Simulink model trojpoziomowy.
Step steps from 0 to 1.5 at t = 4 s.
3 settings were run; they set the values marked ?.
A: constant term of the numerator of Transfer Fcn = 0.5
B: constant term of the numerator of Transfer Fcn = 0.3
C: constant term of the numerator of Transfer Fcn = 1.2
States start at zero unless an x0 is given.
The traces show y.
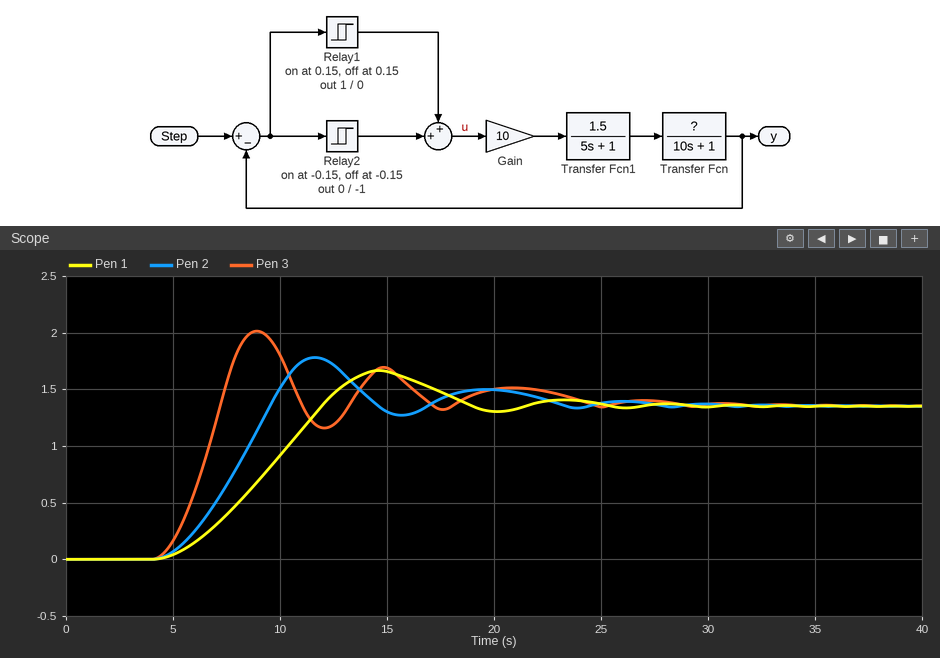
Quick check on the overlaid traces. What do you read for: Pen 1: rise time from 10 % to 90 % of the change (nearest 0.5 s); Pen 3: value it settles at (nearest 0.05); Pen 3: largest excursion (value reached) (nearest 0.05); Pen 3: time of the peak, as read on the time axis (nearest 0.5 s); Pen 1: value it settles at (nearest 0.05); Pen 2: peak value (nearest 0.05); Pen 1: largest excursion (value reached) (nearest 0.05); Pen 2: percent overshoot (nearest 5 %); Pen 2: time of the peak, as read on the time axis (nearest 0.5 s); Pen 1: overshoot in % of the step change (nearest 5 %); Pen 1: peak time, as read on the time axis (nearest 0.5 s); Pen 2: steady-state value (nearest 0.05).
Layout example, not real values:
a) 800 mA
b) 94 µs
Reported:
a) 5.5 s
b) 1.35
c) 2.00
d) 9.0 s
e) 1.35
f) 1.80
g) 1.65
h) 30 %
i) 11.5 s
j) 25 %
k) 14.5 s
l) 1.35
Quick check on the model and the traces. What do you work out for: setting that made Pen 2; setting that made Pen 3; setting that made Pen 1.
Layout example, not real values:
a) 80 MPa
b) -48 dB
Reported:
a) A
b) C
c) B
